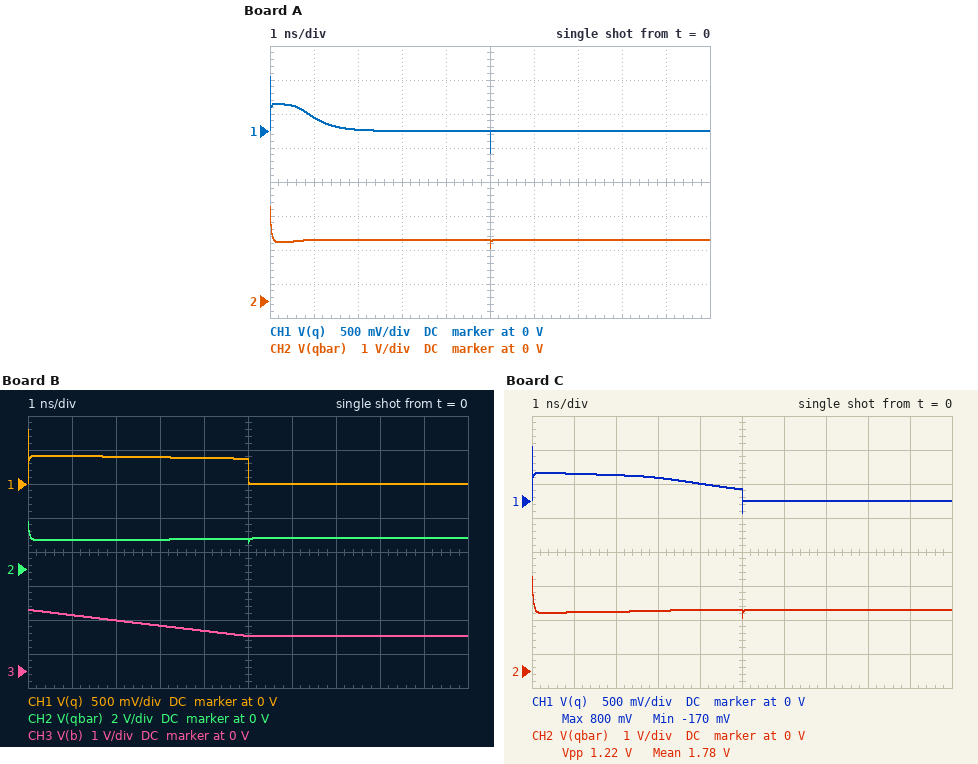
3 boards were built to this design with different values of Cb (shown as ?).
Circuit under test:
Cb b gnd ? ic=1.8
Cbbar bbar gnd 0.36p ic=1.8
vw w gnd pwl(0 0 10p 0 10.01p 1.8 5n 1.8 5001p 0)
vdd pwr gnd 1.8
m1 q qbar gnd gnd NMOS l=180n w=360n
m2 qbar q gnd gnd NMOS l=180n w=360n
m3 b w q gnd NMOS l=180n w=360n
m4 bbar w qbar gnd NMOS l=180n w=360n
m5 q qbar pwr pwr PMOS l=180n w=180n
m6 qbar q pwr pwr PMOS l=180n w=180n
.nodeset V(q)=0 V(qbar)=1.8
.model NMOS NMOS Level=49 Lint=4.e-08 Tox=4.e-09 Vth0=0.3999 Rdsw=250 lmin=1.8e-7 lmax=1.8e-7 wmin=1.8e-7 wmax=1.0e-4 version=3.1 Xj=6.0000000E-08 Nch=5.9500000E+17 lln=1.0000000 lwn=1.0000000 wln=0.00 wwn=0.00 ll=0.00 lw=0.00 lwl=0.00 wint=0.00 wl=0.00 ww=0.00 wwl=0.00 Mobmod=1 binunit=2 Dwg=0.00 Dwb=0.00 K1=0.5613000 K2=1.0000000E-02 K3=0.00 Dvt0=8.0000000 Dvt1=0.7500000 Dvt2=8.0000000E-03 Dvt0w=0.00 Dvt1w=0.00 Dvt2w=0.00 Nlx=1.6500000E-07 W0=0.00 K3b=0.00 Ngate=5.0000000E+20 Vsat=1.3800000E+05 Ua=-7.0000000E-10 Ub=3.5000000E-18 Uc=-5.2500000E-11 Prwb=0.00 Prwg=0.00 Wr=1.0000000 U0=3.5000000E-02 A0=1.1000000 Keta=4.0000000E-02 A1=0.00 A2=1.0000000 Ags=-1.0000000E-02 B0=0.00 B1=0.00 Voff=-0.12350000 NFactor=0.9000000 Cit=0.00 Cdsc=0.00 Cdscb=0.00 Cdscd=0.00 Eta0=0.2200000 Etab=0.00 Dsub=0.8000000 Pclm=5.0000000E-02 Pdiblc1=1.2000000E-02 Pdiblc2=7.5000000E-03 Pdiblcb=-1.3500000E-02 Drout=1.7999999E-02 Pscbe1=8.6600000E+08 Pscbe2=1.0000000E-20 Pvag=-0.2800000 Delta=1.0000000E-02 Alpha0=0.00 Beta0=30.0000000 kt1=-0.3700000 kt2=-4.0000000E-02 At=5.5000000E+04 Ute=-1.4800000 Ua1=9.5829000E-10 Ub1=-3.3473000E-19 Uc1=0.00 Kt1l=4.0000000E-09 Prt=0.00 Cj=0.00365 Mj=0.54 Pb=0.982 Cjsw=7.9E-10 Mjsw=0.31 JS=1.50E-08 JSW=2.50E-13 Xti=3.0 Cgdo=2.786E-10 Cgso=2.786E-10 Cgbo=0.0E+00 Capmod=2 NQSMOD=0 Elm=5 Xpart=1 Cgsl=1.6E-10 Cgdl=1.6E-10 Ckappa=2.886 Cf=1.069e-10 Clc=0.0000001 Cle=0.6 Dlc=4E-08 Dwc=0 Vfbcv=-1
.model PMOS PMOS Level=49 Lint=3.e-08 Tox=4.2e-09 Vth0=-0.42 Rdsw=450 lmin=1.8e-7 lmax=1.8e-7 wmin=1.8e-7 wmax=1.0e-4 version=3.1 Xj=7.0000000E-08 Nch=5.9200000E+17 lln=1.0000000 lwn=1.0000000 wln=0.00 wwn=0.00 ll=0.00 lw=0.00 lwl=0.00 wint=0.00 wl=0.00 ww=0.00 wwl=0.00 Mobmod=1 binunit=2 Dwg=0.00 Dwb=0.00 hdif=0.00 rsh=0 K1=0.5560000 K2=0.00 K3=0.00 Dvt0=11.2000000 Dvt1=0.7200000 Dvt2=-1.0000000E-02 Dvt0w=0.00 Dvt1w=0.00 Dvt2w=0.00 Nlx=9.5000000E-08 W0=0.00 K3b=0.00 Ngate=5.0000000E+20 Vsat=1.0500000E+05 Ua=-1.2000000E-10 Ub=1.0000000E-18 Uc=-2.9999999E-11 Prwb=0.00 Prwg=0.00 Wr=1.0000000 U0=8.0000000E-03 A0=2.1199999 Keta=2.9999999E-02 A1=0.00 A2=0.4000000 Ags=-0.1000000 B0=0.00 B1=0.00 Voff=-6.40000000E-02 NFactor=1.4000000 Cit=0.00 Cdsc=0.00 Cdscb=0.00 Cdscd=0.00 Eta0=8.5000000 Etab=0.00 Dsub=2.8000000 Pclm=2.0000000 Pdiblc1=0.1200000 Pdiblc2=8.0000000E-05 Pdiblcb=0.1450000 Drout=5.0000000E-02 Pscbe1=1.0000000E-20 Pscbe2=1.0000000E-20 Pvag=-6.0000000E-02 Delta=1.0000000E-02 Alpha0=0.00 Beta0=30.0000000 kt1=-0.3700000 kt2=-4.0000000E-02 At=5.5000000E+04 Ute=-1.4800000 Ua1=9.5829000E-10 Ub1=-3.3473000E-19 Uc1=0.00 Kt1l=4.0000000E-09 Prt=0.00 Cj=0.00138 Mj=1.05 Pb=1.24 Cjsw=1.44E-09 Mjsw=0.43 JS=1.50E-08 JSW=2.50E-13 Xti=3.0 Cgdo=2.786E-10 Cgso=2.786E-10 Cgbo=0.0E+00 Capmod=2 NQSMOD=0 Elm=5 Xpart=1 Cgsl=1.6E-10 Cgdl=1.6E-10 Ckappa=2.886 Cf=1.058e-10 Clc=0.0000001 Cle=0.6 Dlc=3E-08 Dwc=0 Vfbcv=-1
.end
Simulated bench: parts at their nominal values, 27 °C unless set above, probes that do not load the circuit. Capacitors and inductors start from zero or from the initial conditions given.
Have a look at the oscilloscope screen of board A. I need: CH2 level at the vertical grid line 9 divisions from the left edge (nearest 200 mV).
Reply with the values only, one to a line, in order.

1.8 V
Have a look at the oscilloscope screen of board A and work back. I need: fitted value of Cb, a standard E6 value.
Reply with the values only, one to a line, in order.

100 fF
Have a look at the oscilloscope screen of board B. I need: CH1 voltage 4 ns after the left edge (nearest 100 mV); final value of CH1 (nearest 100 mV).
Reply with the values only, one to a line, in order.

400 mV
0 V
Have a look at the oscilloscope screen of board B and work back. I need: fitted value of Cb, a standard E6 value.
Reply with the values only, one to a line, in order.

1 pF
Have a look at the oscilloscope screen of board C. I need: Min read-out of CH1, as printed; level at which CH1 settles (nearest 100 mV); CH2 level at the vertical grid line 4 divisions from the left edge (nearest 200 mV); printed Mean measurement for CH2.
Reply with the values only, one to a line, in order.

-170 mV
0 V
1.8 V
1.78 V
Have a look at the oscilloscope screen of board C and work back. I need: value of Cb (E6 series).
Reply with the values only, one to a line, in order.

470 fF
